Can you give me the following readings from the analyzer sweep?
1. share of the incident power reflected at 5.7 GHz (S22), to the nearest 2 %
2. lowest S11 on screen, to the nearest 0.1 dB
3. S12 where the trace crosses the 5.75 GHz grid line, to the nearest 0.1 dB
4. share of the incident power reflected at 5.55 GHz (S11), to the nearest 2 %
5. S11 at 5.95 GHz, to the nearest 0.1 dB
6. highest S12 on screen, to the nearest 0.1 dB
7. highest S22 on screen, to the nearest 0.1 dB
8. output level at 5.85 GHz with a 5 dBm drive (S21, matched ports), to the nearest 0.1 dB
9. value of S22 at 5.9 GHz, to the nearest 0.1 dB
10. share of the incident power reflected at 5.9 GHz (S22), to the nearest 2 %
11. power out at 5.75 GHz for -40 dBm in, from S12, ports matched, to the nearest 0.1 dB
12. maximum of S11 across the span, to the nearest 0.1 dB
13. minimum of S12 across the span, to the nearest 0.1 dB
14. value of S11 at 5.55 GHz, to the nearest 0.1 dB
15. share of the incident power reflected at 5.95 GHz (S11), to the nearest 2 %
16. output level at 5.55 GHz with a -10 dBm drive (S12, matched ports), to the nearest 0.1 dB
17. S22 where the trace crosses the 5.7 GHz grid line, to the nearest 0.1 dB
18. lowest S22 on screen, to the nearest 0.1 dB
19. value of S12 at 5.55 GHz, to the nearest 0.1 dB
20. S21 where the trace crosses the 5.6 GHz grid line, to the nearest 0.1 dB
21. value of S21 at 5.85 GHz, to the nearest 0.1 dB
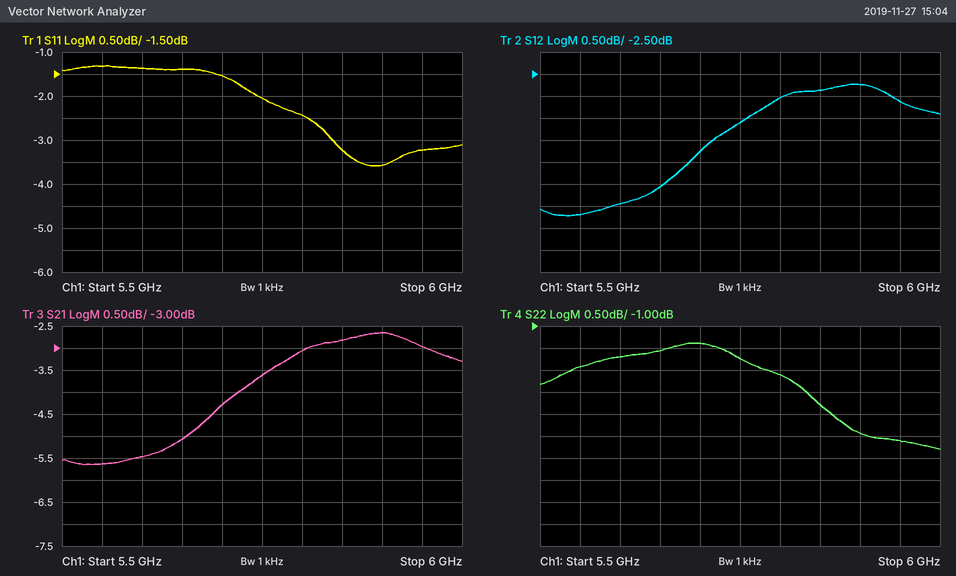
72 %
-3.6 dB
-3.6 dB
74 %
-3.2 dB
-2.7 dB
-1.4 dB
2.2 dBm
-3.4 dB
46 %
-43.6 dBm
-1.3 dB
-5.7 dB
-1.3 dB
48 %
-15.7 dBm
-1.4 dB
-3.8 dB
-5.7 dB
-5.5 dB
-2.8 dB
